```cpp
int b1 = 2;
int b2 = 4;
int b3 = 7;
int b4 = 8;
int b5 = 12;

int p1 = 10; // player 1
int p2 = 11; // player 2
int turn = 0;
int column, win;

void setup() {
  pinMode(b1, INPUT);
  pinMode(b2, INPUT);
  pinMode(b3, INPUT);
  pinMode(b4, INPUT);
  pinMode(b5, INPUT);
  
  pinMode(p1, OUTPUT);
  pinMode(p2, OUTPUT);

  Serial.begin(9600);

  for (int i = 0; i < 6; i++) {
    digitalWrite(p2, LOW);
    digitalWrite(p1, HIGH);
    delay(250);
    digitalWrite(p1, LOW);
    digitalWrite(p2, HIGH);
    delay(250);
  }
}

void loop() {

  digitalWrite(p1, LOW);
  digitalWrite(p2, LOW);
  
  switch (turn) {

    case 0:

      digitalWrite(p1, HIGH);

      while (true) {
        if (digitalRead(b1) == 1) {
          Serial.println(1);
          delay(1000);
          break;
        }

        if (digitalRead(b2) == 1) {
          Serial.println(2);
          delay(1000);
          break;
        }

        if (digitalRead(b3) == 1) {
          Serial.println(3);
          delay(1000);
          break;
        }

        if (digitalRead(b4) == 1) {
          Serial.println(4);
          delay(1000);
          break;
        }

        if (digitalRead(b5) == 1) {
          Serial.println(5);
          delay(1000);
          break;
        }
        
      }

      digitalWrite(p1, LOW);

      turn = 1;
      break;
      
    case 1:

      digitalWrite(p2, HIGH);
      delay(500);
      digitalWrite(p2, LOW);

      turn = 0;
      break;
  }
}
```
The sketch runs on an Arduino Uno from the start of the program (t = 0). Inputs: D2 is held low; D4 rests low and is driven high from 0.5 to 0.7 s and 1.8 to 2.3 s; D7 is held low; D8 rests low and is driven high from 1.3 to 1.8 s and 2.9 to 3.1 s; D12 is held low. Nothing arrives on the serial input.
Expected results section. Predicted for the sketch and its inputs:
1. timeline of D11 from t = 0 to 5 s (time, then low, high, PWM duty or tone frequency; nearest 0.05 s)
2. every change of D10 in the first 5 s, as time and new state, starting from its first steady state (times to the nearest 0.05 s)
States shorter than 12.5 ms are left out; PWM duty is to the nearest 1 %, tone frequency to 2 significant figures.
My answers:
0 s low; 0.25 s high; 0.5 s low; 0.75 s high; 1 s low; 1.25 s high; 1.5 s low; 1.75 s high; 2 s low; 2.25 s high; 2.5 s low; 2.75 s high; 3 s low; 4 s high; 4.5 s low
0 s high; 0.25 s low; 0.5 s high; 0.75 s low; 1 s high; 1.25 s low; 1.5 s high; 1.75 s low; 2 s high; 2.25 s low; 2.5 s high; 2.75 s low; 3 s high; 4 s low; 4.5 s high
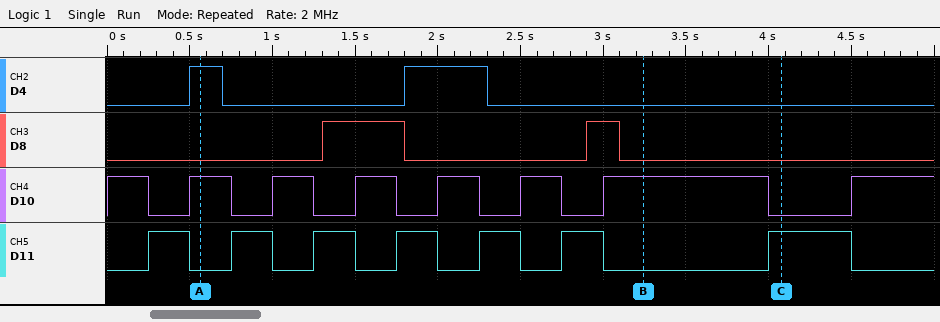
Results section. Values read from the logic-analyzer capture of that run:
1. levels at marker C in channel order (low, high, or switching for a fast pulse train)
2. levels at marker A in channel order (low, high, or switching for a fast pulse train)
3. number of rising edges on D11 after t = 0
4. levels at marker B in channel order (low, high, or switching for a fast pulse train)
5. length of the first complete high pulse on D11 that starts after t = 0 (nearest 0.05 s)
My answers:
D4 low, D8 low, D10 low, D11 high
D4 high, D8 low, D10 high, D11 low
7
D4 low, D8 low, D10 high, D11 low
0.25 s
